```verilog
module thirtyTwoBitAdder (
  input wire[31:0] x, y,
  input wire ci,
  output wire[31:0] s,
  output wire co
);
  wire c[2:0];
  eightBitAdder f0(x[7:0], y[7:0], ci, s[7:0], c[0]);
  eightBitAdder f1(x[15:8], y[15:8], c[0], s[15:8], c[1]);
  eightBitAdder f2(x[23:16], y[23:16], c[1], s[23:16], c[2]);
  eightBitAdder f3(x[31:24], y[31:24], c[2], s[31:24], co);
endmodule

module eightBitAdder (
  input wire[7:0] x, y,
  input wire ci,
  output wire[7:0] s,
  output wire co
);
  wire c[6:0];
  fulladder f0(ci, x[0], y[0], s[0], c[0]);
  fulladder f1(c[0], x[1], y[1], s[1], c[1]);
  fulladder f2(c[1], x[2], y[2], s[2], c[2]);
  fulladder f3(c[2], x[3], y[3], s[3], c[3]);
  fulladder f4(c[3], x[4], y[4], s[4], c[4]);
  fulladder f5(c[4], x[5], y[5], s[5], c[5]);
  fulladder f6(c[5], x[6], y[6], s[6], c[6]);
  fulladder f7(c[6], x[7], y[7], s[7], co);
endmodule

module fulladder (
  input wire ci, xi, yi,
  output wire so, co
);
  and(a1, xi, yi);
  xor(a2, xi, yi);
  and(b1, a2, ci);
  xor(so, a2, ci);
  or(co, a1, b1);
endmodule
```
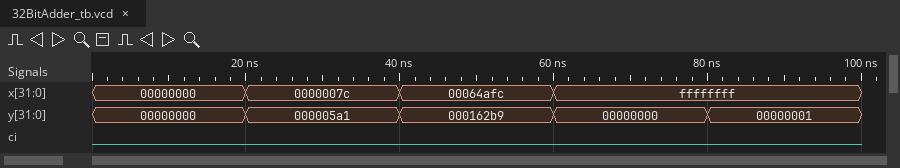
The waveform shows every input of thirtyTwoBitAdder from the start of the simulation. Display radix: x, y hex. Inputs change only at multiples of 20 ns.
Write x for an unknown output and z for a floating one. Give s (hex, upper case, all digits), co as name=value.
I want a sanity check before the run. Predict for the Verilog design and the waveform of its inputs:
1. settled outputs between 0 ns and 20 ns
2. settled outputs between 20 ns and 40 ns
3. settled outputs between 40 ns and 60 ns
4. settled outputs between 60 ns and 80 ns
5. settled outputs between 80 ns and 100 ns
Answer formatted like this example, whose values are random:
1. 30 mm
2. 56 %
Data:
1. s=00000000, co=0
2. s=0000061D, co=0
3. s=0007ADB5, co=0
4. s=FFFFFFFF, co=0
5. s=00000000, co=1
